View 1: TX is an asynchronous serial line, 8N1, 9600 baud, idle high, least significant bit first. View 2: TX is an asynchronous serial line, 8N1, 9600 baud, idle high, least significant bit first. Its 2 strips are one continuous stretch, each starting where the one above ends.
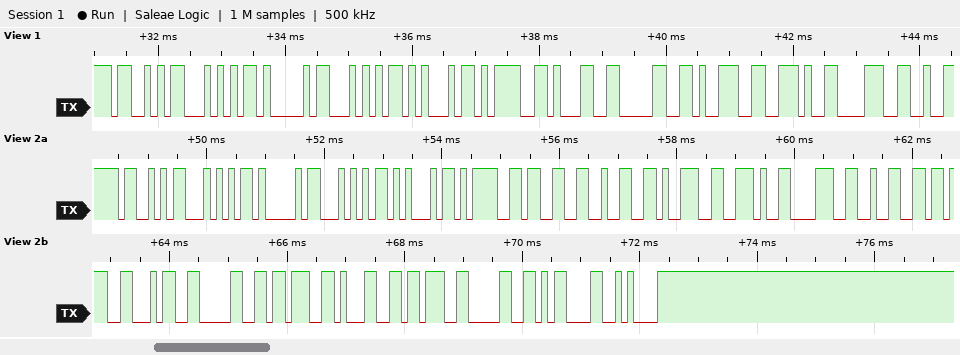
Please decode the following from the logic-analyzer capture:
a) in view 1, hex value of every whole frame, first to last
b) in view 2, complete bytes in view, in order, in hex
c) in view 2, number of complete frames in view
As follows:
53 54 41 54 45 3D 31 30 39 2E 38
53 54 41 54 45 3D 33 32 39 2E 38 32 3B 34 30 3B 31 3B 30 0D 0A
21
